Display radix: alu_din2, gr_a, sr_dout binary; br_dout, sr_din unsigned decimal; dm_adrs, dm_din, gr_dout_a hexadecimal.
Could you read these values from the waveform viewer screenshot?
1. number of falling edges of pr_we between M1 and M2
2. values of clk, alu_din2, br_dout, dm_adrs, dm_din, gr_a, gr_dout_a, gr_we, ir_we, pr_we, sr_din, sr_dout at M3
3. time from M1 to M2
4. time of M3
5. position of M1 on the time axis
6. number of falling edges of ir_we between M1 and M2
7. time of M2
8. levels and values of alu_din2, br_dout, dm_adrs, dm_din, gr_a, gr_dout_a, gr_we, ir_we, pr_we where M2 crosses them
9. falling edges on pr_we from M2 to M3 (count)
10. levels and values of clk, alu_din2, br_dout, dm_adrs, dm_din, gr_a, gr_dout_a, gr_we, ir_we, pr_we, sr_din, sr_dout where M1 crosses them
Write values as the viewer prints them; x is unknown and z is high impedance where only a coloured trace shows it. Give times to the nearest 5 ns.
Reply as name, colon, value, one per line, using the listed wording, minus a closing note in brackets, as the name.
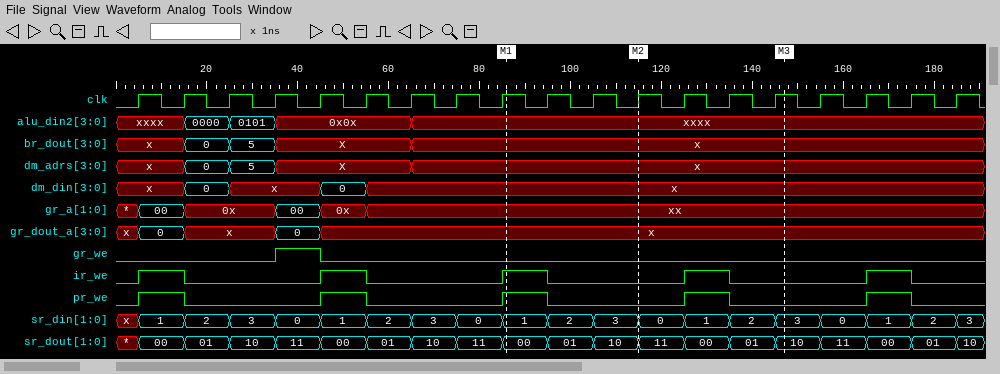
number of falling edges of pr_we between M1 and M2: 1
values of clk, alu_din2, br_dout, dm_adrs, dm_din, gr_a, gr_dout_a, gr_we, ir_we, pr_we, sr_din, sr_dout at M3: clk=1, alu_din2=xxxx, br_dout=x, dm_adrs=x, dm_din=x, gr_a=xx, gr_dout_a=x, gr_we=0, ir_we=0, pr_we=0, sr_din=3, sr_dout=10
time from M1 to M2: 30 ns
time of M3: 145 ns
position of M1 on the time axis: 85 ns
number of falling edges of ir_we between M1 and M2: 1
time of M2: 115 ns
levels and values of alu_din2, br_dout, dm_adrs, dm_din, gr_a, gr_dout_a, gr_we, ir_we, pr_we where M2 crosses them: alu_din2=xxxx, br_dout=x, dm_adrs=x, dm_din=x, gr_a=xx, gr_dout_a=x, gr_we=0, ir_we=0, pr_we=0
falling edges on pr_we from M2 to M3: 1
levels and values of clk, alu_din2, br_dout, dm_adrs, dm_din, gr_a, gr_dout_a, gr_we, ir_we, pr_we, sr_din, sr_dout where M1 crosses them: clk=1, alu_din2=xxxx, br_dout=x, dm_adrs=x, dm_din=x, gr_a=xx, gr_dout_a=x, gr_we=0, ir_we=1, pr_we=1, sr_din=1, sr_dout=00
